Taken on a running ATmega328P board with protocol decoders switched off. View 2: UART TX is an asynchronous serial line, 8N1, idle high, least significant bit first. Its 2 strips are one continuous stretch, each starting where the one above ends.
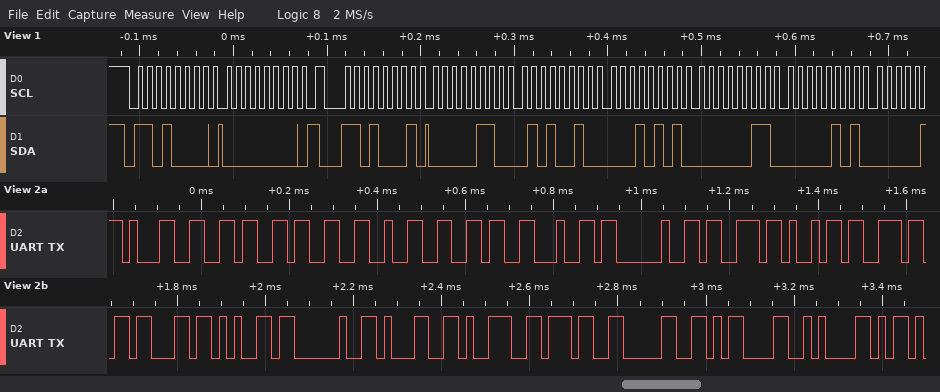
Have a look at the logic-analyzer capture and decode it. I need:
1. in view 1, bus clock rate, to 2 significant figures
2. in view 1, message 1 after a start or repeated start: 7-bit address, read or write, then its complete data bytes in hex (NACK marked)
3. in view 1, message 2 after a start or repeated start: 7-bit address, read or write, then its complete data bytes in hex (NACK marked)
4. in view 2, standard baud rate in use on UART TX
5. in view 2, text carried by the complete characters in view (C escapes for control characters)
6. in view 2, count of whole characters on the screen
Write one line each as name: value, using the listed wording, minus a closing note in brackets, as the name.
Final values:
in view 1, bus clock rate, to 2 significant figures: 100 kHz
in view 1, message 1 after a start or repeated start: 7-bit address, read or write, then its complete data bytes in hex: 0x68 write: 00
in view 1, message 2 after a start or repeated start: 7-bit address, read or write, then its complete data bytes in hex: 0x68 read: 06 52 15 03 05
in view 2, standard baud rate in use on UART TX: 57600 baud
in view 2, text carried by the complete characters in view: "16326d since 1970\r\n"
in view 2, count of whole characters on the screen: 19
